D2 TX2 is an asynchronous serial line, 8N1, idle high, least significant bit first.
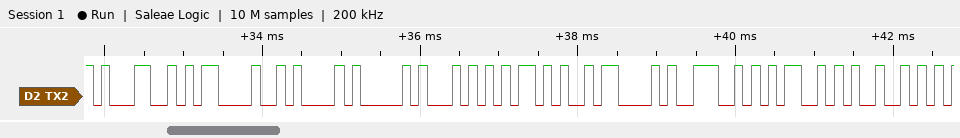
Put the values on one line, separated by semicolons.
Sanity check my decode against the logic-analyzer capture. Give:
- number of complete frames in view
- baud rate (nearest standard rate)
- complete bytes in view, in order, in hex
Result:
10; 9600 baud; 0x31 0x0D 0x0A 0x41 0x54 0x2B 0x43 0x4E 0x4D 0x49
